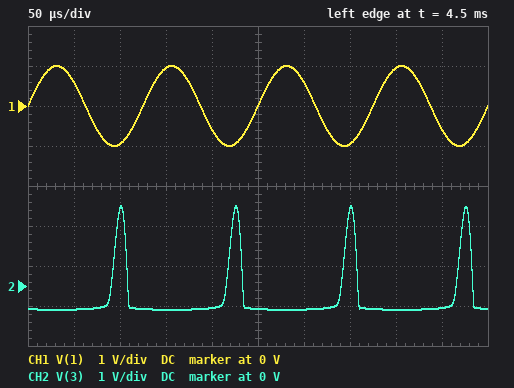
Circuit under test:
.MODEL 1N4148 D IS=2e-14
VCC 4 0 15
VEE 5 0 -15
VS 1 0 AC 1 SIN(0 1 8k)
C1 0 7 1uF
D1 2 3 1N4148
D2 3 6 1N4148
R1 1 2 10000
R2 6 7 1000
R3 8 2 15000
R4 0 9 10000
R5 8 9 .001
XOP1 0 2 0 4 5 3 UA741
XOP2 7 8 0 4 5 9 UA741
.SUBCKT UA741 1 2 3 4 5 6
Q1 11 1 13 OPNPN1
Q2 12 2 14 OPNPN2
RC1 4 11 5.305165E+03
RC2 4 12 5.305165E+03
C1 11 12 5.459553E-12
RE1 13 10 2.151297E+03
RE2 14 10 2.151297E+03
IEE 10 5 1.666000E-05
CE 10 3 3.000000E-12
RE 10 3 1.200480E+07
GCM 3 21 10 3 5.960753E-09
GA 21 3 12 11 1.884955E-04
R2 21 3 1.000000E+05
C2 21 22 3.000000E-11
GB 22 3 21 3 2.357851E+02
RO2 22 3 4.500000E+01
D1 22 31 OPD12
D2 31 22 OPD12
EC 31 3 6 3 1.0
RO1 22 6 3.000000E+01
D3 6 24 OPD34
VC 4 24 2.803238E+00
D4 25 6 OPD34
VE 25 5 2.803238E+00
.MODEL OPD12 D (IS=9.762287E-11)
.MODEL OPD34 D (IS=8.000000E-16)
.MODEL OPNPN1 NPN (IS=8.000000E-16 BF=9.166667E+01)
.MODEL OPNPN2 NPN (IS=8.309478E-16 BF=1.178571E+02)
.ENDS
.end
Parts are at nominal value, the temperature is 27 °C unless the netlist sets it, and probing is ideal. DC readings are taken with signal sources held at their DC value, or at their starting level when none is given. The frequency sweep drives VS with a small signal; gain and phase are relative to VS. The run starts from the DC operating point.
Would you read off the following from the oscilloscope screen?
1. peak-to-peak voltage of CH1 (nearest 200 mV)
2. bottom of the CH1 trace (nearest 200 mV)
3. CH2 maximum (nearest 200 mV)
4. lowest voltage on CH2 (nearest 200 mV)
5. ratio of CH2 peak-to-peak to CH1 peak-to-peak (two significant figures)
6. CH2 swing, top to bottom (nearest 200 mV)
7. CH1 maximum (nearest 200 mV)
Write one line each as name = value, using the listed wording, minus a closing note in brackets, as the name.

peak-to-peak voltage of CH1 = 2.0 V
bottom of the CH1 trace = -1.0 V
CH2 maximum = 2.0 V
lowest voltage on CH2 = -600 mV
ratio of CH2 peak-to-peak to CH1 peak-to-peak = 1.3
CH2 swing, top to bottom = 2.6 V
CH1 maximum = 1.0 V
